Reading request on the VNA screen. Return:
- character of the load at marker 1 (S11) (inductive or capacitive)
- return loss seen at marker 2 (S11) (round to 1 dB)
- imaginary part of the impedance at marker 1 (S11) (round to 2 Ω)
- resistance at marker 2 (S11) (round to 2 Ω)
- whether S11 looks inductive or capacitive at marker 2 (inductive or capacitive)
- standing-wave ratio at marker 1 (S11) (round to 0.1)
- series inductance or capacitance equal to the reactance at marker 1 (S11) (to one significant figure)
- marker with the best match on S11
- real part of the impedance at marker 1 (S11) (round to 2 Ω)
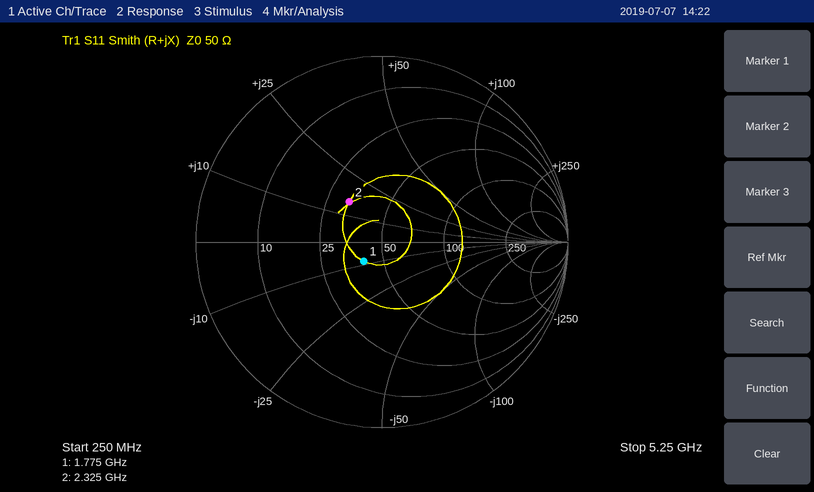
capacitive
11 dB
-8 Ω
32 Ω
inductive
1.3
10 pF
marker 1
40 Ω
